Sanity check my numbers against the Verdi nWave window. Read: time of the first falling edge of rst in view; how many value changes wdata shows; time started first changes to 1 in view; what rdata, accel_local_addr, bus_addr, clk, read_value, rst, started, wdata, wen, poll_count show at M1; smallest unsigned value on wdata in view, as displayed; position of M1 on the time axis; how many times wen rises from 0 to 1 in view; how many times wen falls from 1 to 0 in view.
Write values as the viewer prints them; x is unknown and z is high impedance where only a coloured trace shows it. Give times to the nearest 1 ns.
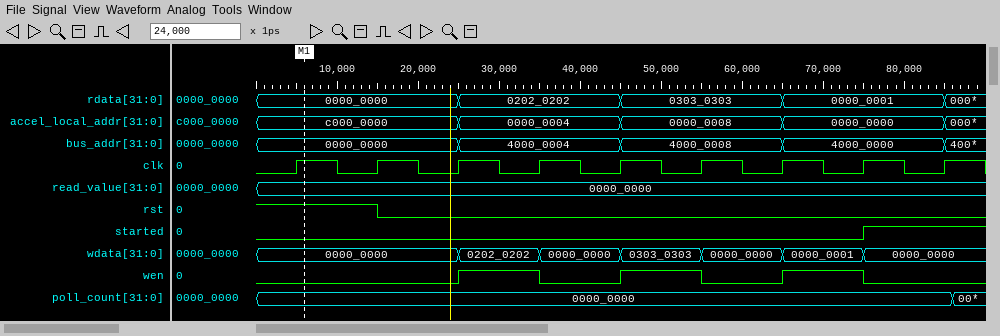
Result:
15 ns
6
75 ns
rdata=0000_0000, accel_local_addr=c000_0000, bus_addr=0000_0000, clk=1, read_value=0000_0000, rst=1, started=0, wdata=0000_0000, wen=0, poll_count=0000_0000
0000_0000
6 ns
3
3
